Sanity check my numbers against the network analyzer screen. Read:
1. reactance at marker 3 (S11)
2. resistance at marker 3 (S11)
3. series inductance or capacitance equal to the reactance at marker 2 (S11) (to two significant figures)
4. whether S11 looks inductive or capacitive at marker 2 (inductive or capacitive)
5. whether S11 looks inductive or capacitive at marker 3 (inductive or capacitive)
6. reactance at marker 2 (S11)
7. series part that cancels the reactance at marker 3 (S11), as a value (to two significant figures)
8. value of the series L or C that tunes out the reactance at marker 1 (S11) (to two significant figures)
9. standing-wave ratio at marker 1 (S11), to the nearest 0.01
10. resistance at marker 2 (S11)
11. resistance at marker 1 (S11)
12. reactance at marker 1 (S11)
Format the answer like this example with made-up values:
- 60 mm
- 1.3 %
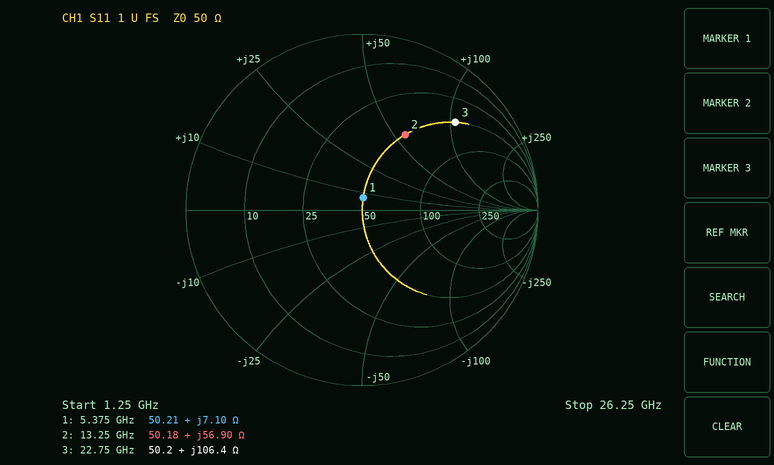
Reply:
- +106.4 Ω
- 50.2 Ω
- 680 pH
- inductive
- inductive
- +56.90 Ω
- 66 fF
- 4.2 pF
- 1.15
- 50.18 Ω
- 50.21 Ω
- +7.10 Ω
